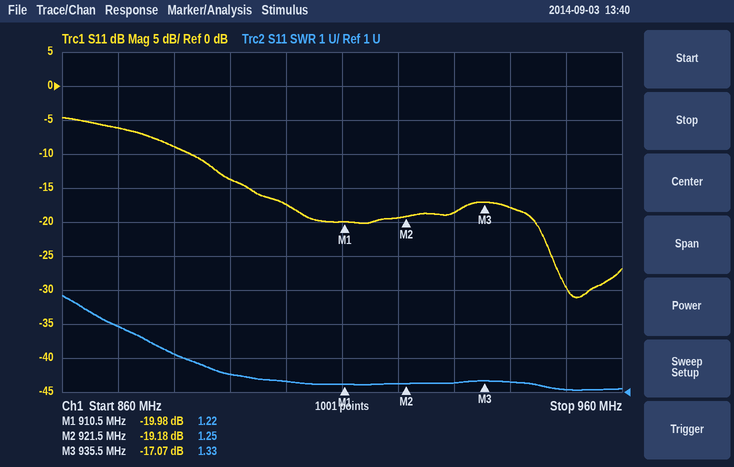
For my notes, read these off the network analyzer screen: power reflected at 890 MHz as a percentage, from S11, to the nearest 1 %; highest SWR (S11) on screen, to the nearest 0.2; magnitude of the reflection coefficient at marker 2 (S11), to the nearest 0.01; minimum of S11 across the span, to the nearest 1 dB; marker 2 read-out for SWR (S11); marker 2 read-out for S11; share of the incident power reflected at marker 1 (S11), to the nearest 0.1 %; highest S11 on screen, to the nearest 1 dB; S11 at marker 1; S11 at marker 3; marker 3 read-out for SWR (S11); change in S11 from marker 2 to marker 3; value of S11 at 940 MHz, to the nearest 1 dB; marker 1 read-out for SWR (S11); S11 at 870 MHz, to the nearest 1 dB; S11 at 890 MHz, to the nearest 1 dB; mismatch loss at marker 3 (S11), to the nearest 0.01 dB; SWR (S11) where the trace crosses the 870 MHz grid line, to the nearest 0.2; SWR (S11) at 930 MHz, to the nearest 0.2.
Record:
4 %
3.8
0.11
-31 dB
1.25
-19.18 dB
1.0 %
-5 dB
-19.98 dB
-17.07 dB
1.33
2.11 dB
-18 dB
1.22
-6 dB
-14 dB
0.09 dB
3.0
1.2
